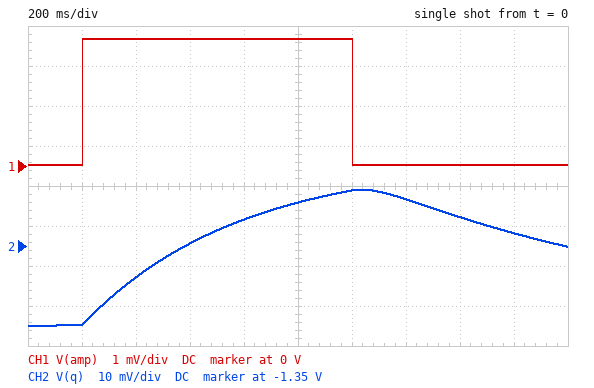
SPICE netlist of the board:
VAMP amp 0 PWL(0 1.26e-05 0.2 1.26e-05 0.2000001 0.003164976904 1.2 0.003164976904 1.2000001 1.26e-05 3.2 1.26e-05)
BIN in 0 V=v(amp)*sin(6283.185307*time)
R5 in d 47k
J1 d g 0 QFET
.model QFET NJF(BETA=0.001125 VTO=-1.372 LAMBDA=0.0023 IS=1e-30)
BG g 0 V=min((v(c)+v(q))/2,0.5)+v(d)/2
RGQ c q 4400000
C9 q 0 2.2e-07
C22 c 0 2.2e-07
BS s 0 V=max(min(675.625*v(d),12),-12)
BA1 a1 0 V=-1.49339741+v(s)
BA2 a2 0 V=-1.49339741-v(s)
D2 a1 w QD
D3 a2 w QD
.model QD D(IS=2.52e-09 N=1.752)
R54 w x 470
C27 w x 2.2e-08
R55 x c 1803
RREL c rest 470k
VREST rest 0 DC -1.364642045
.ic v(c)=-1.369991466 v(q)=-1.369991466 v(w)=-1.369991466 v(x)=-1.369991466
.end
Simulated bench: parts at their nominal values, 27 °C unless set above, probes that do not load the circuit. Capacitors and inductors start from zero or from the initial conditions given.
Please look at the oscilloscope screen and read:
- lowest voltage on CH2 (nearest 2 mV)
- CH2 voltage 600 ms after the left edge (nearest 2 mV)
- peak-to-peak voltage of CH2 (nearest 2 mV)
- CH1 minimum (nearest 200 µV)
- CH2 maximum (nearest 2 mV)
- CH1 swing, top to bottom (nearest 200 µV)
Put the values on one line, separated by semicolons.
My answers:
-1.370 V; -1.350 V; 34 mV; 0 V; -1.336 V; 3.2 mV
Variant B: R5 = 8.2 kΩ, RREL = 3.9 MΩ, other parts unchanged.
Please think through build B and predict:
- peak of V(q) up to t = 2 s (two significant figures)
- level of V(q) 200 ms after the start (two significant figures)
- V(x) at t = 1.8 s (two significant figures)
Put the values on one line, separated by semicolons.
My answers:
-1.2 V; -1.4 V; -1.3 V
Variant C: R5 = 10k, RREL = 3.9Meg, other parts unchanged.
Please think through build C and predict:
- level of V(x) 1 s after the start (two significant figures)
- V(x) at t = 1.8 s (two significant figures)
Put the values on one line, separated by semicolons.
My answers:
-1.2 V; -1.3 V
